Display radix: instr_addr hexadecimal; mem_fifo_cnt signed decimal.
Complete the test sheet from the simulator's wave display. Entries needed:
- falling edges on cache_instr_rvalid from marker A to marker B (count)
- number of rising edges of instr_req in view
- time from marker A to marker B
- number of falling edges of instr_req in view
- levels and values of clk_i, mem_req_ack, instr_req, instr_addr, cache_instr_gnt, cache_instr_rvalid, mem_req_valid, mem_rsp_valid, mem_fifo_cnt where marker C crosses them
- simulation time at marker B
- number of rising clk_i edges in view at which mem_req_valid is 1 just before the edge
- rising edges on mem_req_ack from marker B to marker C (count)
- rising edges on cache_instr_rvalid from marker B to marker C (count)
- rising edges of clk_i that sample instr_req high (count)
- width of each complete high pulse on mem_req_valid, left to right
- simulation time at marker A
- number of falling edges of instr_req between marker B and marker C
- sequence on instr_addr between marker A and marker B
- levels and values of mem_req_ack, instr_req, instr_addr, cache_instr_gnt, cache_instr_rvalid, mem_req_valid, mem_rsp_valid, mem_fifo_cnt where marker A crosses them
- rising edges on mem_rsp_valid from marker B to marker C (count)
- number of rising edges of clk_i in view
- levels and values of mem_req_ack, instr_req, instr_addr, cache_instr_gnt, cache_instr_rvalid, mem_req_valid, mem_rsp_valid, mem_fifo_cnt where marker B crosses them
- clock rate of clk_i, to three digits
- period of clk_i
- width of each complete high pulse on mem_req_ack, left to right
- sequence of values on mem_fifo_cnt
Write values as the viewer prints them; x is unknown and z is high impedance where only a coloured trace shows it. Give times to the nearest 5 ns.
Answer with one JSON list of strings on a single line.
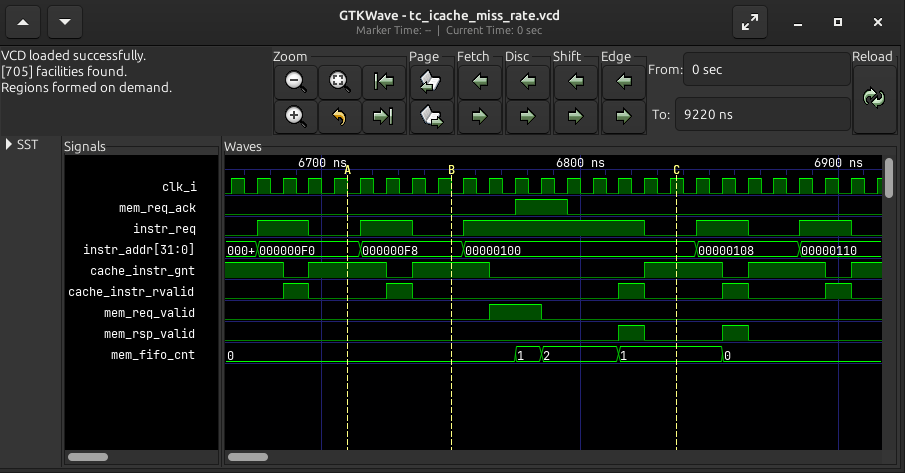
["1", "5", "40 ns", "5", "clk_i=1, mem_req_ack=0, instr_req=0, instr_addr=00000100, cache_instr_gnt=1, cache_instr_rvalid=0, mem_req_valid=0, mem_rsp_valid=0, mem_fifo_cnt=1", "6750 ns", "2", "1", "1", "15", "20 ns", "6710 ns", "1", "000000F0, 000000F8", "mem_req_ack=0, instr_req=0, instr_addr=000000F0, cache_instr_gnt=1, cache_instr_rvalid=0, mem_req_valid=0, mem_rsp_valid=0, mem_fifo_cnt=0", "1", "26", "mem_req_ack=0, instr_req=0, instr_addr=000000F8, cache_instr_gnt=1, cache_instr_rvalid=0, mem_req_valid=0, mem_rsp_valid=0, mem_fifo_cnt=0", "100 MHz", "10 ns", "20 ns", "0, 1, 2, 1, 0"]
